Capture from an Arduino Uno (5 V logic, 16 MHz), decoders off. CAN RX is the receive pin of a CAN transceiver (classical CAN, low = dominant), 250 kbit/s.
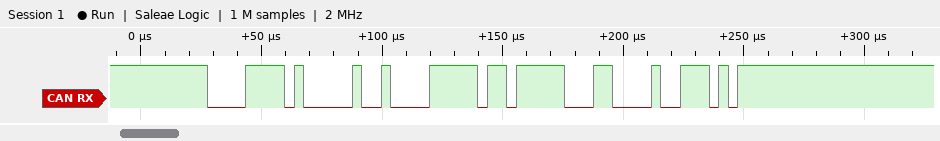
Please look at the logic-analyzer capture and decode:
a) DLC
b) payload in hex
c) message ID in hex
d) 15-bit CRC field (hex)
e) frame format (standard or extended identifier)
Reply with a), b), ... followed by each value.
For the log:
a) 2
b) 1F DF
c) 0x0F4
d) 0x184E
e) standard
